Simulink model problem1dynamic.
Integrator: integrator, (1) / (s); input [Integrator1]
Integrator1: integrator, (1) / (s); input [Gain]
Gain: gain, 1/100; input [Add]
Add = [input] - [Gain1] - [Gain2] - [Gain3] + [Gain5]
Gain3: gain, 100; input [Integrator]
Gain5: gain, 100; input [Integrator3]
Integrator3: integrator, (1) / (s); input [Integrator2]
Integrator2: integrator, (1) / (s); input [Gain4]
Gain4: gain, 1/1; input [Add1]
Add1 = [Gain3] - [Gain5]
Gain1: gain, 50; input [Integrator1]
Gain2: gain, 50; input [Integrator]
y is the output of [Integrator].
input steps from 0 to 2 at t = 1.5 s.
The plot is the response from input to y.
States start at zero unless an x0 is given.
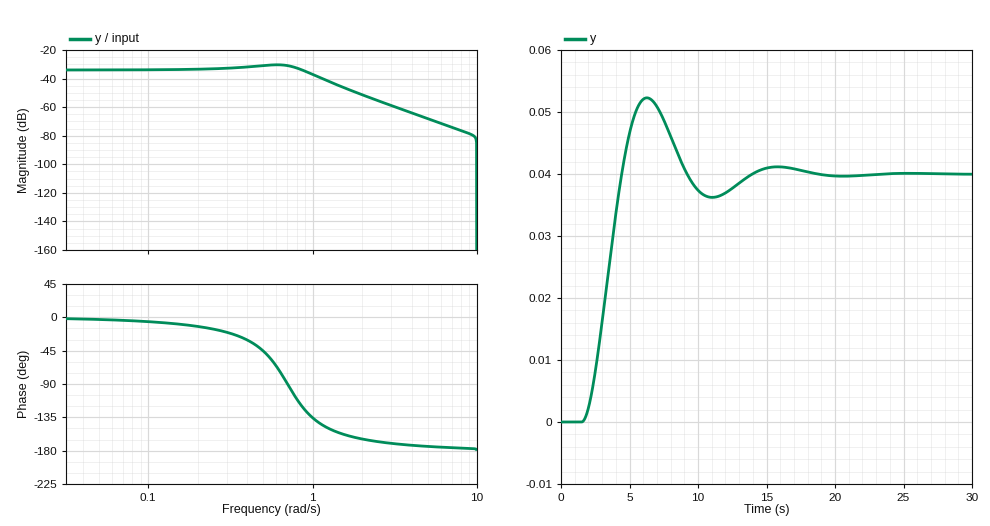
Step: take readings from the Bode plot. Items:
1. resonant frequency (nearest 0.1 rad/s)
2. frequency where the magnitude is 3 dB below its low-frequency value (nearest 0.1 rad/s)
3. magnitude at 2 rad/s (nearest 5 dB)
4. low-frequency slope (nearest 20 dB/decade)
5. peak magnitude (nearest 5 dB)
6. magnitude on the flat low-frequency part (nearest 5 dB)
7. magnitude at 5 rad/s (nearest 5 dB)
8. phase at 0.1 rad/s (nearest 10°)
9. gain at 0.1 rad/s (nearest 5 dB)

0.6 rad/s
1.0 rad/s
-50 dB
0 dB/decade
-30 dB
-35 dB
-70 dB
-10°
-35 dB
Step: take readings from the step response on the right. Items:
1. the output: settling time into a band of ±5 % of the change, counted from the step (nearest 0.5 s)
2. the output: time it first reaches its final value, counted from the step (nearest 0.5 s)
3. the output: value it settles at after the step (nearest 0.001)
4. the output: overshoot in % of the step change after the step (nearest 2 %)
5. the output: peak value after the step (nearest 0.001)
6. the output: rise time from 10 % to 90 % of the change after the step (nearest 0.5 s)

11.0 s
3.0 s
0.040
30 %
0.052
2.0 s
